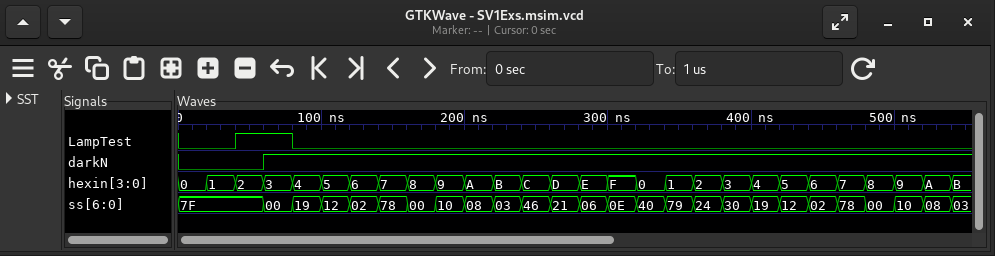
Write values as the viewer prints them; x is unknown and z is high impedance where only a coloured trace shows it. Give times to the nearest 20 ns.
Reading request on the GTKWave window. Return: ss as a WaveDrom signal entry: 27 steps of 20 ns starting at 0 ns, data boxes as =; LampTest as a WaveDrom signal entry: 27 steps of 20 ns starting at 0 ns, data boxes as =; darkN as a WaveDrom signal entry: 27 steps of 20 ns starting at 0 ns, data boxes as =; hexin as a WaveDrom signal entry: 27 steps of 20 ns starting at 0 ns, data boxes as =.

{name: 'ss', wave: '=..========================', data: '7F 00 19 12 02 78 00 10 08 03 46 21 06 0E 40 79 24 30 19 12 02 78 00 10 08'}
{name: 'LampTest', wave: '0.1.0......................'}
{name: 'darkN', wave: '0..1.......................'}
{name: 'hexin', wave: '===========================', data: '0 1 2 3 4 5 6 7 8 9 A B C D E F 0 1 2 3 4 5 6 7 8 9 A'}
